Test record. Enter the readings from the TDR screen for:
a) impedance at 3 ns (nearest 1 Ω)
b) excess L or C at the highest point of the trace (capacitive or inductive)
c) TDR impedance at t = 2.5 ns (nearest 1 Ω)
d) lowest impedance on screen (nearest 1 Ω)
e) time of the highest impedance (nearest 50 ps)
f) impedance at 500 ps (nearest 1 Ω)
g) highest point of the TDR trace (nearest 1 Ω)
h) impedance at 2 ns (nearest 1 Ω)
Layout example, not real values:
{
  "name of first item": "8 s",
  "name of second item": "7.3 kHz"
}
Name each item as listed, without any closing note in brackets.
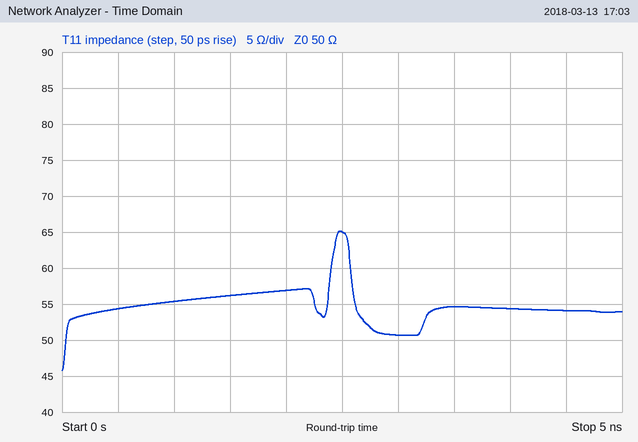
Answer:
{
  "impedance at 3 ns": "51 Ω",
  "excess L or C at the highest point of the trace": "inductive",
  "TDR impedance at t = 2.5 ns": "65 Ω",
  "lowest impedance on screen": "46 Ω",
  "time of the highest impedance": "2.50 ns",
  "impedance at 500 ps": "54 Ω",
  "highest point of the TDR trace": "65 Ω",
  "impedance at 2 ns": "57 Ω"
}
